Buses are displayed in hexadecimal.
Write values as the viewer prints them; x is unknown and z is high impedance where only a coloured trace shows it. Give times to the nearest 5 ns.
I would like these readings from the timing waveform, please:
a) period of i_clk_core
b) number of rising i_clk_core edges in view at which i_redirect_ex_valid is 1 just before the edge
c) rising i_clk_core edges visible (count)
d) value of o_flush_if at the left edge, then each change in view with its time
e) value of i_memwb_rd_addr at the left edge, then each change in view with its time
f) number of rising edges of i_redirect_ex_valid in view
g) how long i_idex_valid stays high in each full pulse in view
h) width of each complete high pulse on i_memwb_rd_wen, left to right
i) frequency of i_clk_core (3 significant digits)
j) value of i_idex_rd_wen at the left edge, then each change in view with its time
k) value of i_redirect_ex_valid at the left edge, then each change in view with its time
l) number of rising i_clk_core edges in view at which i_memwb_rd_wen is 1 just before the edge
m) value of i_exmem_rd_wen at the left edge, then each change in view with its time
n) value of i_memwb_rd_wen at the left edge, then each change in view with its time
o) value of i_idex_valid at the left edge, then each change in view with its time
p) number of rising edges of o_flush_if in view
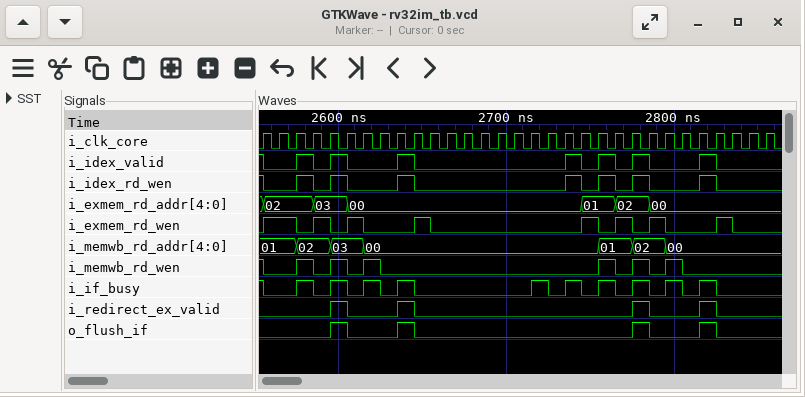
10 ns
4
31
0, 1 at 2595 ns, 0 at 2605 ns, 1 at 2635 ns, 0 at 2645 ns, 1 at 2775 ns, 0 at 2785 ns, 1 at 2815 ns, 0 at 2825 ns
01, 02 at 2575 ns, 03 at 2595 ns, 00 at 2615 ns, 01 at 2755 ns, 02 at 2775 ns, 00 at 2795 ns
4
10 ns, 10 ns, 10 ns, 10 ns, 10 ns, 10 ns, 10 ns
10 ns, 10 ns, 10 ns, 10 ns, 10 ns, 10 ns
100 MHz
1, 0 at 2555 ns, 1 at 2575 ns, 0 at 2585 ns, 1 at 2595 ns, 0 at 2605 ns, 1 at 2635 ns, 0 at 2645 ns, 1 at 2735 ns, 0 at 2745 ns, 1 at 2755 ns, 0 at 2765 ns, 1 at 2775 ns, 0 at 2785 ns, 1 at 2815 ns, 0 at 2825 ns
0, 1 at 2595 ns, 0 at 2605 ns, 1 at 2635 ns, 0 at 2645 ns, 1 at 2775 ns, 0 at 2785 ns, 1 at 2815 ns, 0 at 2825 ns
7
0, 1 at 2555 ns, 0 at 2575 ns, 1 at 2585 ns, 0 at 2595 ns, 1 at 2605 ns, 0 at 2615 ns, 1 at 2645 ns, 0 at 2655 ns, 1 at 2745 ns, 0 at 2755 ns, 1 at 2765 ns, 0 at 2775 ns, 1 at 2785 ns, 0 at 2795 ns, 1 at 2825 ns, 0 at 2835 ns
1, 0 at 2555 ns, 1 at 2575 ns, 0 at 2585 ns, 1 at 2595 ns, 0 at 2605 ns, 1 at 2615 ns, 0 at 2625 ns, 1 at 2755 ns, 0 at 2765 ns, 1 at 2775 ns, 0 at 2785 ns, 1 at 2795 ns, 0 at 2805 ns
1, 0 at 2555 ns, 1 at 2575 ns, 0 at 2585 ns, 1 at 2595 ns, 0 at 2605 ns, 1 at 2635 ns, 0 at 2645 ns, 1 at 2735 ns, 0 at 2745 ns, 1 at 2755 ns, 0 at 2765 ns, 1 at 2775 ns, 0 at 2785 ns, 1 at 2815 ns, 0 at 2825 ns
4
